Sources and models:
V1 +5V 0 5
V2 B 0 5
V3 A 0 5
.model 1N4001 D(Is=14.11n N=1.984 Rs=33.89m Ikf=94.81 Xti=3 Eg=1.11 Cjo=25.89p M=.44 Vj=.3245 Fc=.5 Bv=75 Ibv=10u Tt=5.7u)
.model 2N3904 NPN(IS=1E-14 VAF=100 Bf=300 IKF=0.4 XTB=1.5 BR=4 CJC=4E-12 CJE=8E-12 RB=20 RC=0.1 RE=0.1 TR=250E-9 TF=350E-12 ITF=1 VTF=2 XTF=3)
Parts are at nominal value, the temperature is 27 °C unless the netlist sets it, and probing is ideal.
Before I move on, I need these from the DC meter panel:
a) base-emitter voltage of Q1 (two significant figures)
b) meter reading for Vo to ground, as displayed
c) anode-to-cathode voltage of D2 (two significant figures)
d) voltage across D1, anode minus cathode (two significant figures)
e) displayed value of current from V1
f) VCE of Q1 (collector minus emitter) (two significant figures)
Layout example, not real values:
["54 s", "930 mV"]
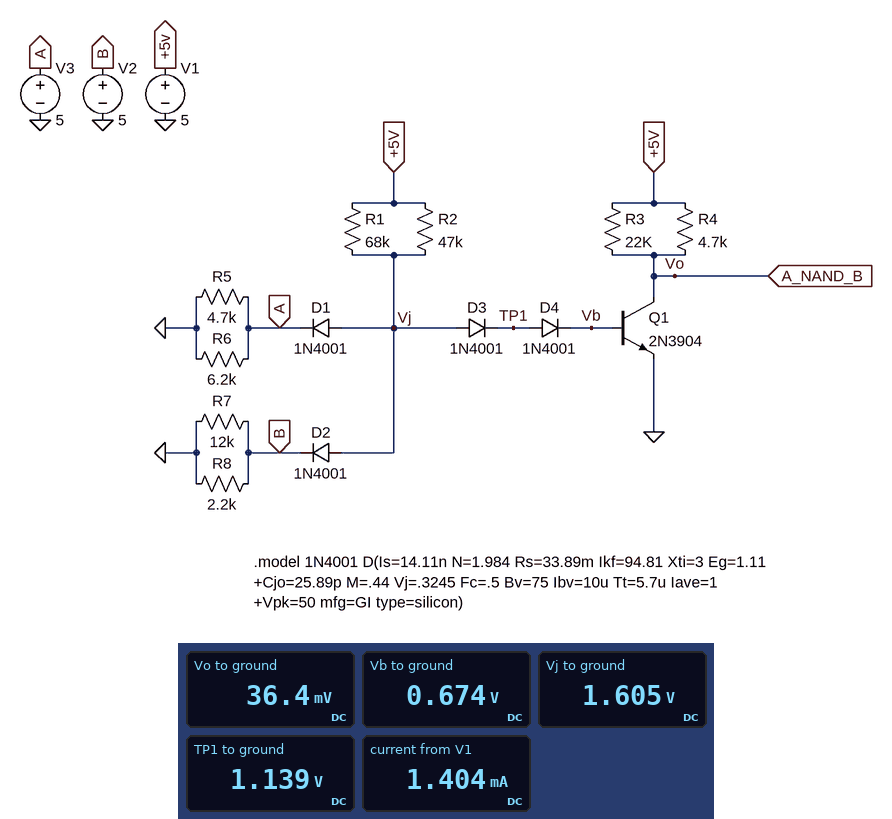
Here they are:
["670 mV", "36.4 mV", "-3.4 V", "-3.4 V", "1.404 mA", "36 mV"]
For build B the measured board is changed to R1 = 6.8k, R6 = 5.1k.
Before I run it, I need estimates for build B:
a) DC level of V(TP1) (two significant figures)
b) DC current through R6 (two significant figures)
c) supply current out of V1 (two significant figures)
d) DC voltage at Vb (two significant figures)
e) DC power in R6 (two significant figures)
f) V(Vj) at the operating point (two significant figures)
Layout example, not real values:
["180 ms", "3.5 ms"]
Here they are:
["1.2 V", "980 µA", "1.8 mA", "700 mV", "4.9 mW", "1.8 V"]
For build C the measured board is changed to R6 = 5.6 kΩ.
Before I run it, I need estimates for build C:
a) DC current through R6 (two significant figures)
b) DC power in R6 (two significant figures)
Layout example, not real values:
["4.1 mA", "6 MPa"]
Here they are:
["890 µA", "4.5 mW"]
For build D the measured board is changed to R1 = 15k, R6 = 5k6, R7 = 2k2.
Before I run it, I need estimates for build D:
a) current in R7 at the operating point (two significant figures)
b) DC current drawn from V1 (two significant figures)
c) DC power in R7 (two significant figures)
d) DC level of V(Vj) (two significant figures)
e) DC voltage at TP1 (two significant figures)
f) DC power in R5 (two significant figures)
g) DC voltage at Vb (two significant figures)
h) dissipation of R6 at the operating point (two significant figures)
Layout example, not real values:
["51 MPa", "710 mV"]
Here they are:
["2.3 mA", "1.6 mA", "11 mW", "1.7 V", "1.2 V", "5.3 mW", "690 mV", "4.5 mW"]
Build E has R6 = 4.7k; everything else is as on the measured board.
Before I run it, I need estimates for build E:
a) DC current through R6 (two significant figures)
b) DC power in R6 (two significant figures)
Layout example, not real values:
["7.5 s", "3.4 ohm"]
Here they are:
["1.1 mA", "5.3 mW"]
